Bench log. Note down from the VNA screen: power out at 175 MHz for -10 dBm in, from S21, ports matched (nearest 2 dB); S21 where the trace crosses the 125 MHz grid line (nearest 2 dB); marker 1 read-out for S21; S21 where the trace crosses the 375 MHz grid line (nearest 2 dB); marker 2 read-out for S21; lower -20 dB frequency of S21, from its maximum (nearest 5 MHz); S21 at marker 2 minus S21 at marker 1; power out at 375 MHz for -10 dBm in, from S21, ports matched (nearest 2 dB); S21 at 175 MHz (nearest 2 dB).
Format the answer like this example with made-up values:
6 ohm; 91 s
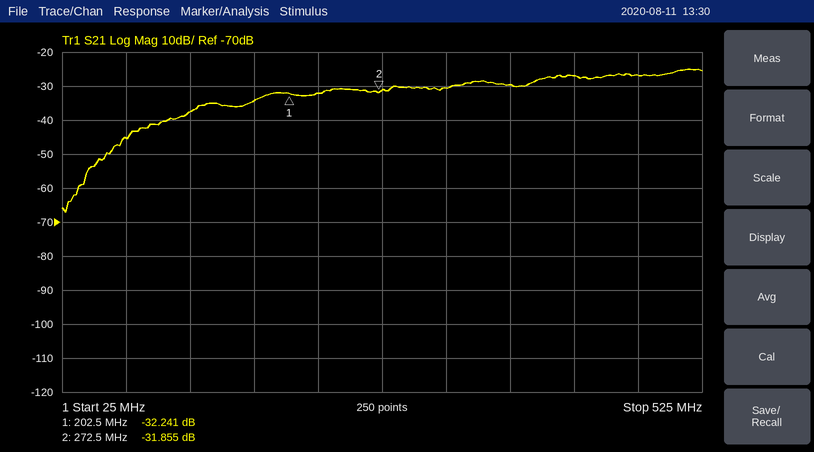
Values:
-44 dBm; -38 dB; -32.241 dB; -30 dB; -31.855 dB; 75 MHz; 0.386 dB; -40 dBm; -34 dB
